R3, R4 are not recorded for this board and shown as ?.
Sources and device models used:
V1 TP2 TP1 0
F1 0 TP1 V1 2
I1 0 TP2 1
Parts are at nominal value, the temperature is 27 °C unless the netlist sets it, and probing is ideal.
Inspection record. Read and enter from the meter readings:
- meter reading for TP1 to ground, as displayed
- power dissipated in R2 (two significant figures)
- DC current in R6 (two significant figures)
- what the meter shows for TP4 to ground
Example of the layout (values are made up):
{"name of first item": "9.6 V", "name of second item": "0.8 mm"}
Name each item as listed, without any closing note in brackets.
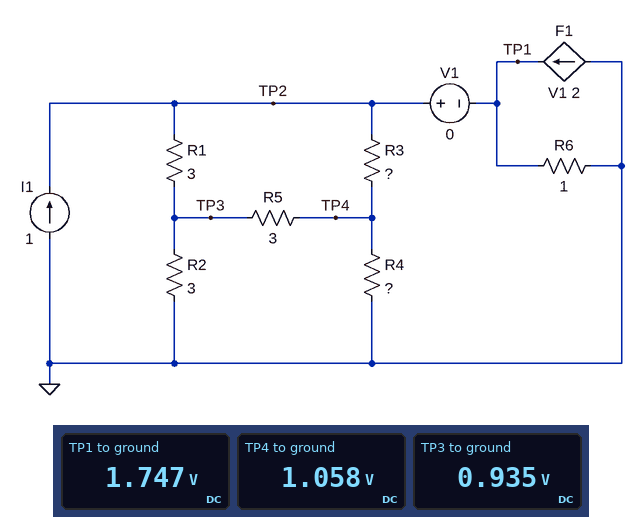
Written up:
{"meter reading for TP1 to ground, as displayed": "1.747 V", "power dissipated in R2": "290 mW", "DC current in R6": "1.7 A", "what the meter shows for TP4 to ground": "1.058 V"}
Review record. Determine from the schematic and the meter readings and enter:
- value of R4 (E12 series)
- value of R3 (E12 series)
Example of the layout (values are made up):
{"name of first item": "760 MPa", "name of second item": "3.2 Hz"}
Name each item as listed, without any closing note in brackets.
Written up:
{"value of R4": "10 Ω", "value of R3": "4.7 Ω"}
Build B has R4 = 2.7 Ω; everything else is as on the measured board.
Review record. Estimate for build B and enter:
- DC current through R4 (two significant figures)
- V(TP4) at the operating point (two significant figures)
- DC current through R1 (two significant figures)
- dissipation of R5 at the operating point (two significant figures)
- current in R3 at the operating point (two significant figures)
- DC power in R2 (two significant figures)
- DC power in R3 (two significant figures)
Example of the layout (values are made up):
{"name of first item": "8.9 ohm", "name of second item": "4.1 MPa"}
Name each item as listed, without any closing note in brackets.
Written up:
{"DC current through R4": "230 mA", "V(TP4) at the operating point": "630 mV", "DC current through R1": "280 mA", "dissipation of R5 at the operating point": "3.5 mW", "current in R3 at the operating point": "200 mA", "DC power in R2": "180 mW", "DC power in R3": "190 mW"}
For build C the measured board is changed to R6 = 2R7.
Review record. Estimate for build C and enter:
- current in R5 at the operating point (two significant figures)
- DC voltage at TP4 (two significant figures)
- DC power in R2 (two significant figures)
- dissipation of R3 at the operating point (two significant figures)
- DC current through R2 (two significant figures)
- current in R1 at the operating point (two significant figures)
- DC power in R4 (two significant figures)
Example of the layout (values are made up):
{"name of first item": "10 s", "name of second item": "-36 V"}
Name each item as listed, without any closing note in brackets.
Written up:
{"current in R5 at the operating point": "65 mA", "DC voltage at TP4": "1.7 V", "DC power in R2": "730 mW", "dissipation of R3 at the operating point": "250 mW", "DC current through R2": "490 mA", "current in R1 at the operating point": "430 mA", "DC power in R4": "280 mW"}
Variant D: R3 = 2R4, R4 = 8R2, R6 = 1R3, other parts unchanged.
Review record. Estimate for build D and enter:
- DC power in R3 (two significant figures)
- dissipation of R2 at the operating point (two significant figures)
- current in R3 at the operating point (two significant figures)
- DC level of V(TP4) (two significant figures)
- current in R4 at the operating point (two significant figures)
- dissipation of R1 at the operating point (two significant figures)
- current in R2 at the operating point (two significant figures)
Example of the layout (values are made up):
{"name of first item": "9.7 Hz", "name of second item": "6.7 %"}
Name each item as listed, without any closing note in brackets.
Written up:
{"DC power in R3": "140 mW", "dissipation of R2 at the operating point": "380 mW", "current in R3 at the operating point": "240 mA", "DC level of V(TP4)": "1.3 V", "current in R4 at the operating point": "160 mA", "dissipation of R1 at the operating point": "230 mW", "current in R2 at the operating point": "360 mA"}
